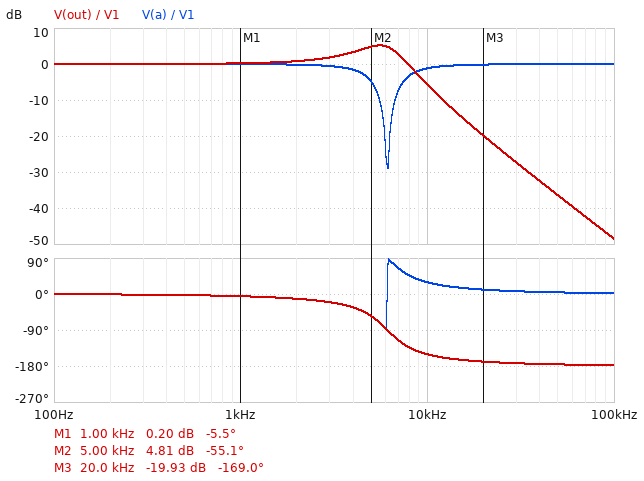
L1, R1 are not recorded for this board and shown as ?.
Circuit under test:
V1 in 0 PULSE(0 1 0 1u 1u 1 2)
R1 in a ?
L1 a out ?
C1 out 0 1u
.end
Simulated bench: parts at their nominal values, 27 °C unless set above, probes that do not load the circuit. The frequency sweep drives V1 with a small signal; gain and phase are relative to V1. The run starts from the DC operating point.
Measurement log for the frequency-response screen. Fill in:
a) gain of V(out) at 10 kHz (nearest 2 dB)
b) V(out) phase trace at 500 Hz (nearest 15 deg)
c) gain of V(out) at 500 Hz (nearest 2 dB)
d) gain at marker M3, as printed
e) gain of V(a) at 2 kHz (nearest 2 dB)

-6 dB
0 deg
0 dB
-19.93 dB
0 dB
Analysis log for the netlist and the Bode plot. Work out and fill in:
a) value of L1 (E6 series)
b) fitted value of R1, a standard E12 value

680 µH
15 Ω
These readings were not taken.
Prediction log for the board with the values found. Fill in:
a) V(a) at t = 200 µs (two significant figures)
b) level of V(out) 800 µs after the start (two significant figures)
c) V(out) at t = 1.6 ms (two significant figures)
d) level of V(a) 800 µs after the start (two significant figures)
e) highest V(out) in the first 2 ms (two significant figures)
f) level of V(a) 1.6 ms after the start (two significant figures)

940 mV
1.0 V
1.0 V
1.0 V
1.4 V
1.0 V
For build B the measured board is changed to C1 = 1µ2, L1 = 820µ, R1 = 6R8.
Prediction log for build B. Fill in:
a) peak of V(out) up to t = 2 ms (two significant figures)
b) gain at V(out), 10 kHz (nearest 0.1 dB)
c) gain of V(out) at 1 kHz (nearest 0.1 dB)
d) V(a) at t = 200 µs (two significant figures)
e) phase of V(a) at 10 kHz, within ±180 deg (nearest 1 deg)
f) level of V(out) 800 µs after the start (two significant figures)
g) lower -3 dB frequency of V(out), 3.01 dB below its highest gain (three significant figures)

1.7 V
-9.3 dB
0.3 dB
1.0 V
10 deg
960 mV
4.27 kHz
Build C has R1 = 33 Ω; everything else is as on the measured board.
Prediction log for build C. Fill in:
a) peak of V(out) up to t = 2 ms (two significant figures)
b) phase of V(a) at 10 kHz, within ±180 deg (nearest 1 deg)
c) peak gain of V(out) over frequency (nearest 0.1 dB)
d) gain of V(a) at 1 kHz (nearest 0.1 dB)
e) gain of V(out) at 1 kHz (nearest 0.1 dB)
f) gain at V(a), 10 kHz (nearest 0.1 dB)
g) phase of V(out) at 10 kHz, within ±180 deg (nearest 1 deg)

1.1 V
51 deg
0.2 dB
-0.2 dB
0 dB
-4.0 dB
-129 deg
